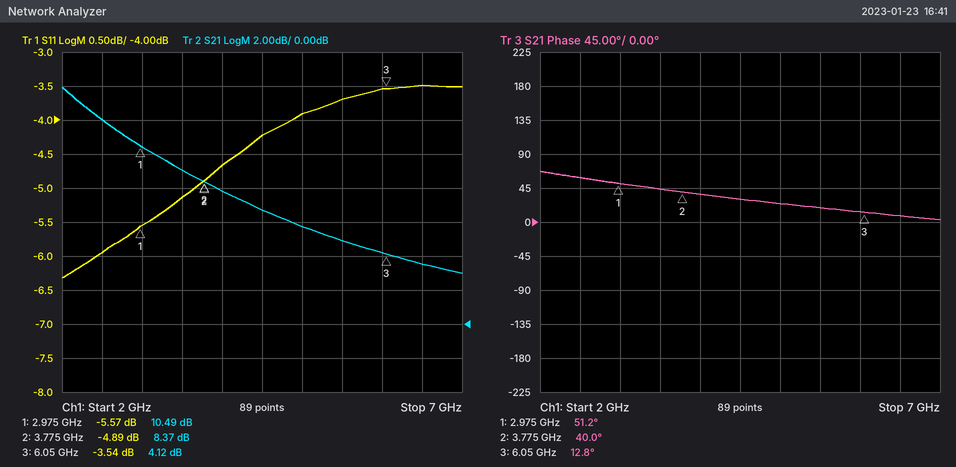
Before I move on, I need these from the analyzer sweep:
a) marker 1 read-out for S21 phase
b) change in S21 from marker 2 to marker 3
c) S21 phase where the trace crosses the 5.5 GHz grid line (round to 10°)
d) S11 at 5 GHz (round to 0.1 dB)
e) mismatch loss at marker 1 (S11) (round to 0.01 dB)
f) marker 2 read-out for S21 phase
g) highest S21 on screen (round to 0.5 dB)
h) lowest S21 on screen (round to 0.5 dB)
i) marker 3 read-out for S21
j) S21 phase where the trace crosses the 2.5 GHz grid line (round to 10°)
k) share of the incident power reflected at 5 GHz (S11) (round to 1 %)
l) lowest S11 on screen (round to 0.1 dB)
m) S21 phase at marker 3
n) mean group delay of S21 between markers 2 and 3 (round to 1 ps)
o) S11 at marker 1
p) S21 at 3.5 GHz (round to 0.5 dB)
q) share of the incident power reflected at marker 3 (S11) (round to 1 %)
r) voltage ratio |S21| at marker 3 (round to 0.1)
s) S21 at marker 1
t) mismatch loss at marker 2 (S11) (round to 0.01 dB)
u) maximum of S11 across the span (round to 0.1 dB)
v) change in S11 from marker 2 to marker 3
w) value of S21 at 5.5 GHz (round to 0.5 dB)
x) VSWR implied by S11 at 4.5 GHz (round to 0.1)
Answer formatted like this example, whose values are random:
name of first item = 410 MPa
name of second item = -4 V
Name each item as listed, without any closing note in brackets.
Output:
marker 1 read-out for S21 phase = 51.2°
change in S21 from marker 2 to marker 3 = -4.25 dB
S21 phase where the trace crosses the 5.5 GHz grid line = 20°
S11 at 5 GHz = -3.9 dB
mismatch loss at marker 1 (S11) = 1.41 dB
marker 2 read-out for S21 phase = 40.0°
highest S21 on screen = 14.0 dB
lowest S21 on screen = 3.0 dB
marker 3 read-out for S21 = 4.12 dB
S21 phase where the trace crosses the 2.5 GHz grid line = 60°
share of the incident power reflected at 5 GHz (S11) = 41 %
lowest S11 on screen = -6.3 dB
S21 phase at marker 3 = 12.8°
mean group delay of S21 between markers 2 and 3 = 33 ps
S11 at marker 1 = -5.57 dB
S21 at 3.5 GHz = 9.0 dB
share of the incident power reflected at marker 3 (S11) = 44 %
voltage ratio |S21| at marker 3 = 1.6
S21 at marker 1 = 10.49 dB
mismatch loss at marker 2 (S11) = 1.70 dB
maximum of S11 across the span = -3.5 dB
change in S11 from marker 2 to marker 3 = 1.35 dB
value of S21 at 5.5 GHz = 5.0 dB
VSWR implied by S11 at 4.5 GHz = 4.2
